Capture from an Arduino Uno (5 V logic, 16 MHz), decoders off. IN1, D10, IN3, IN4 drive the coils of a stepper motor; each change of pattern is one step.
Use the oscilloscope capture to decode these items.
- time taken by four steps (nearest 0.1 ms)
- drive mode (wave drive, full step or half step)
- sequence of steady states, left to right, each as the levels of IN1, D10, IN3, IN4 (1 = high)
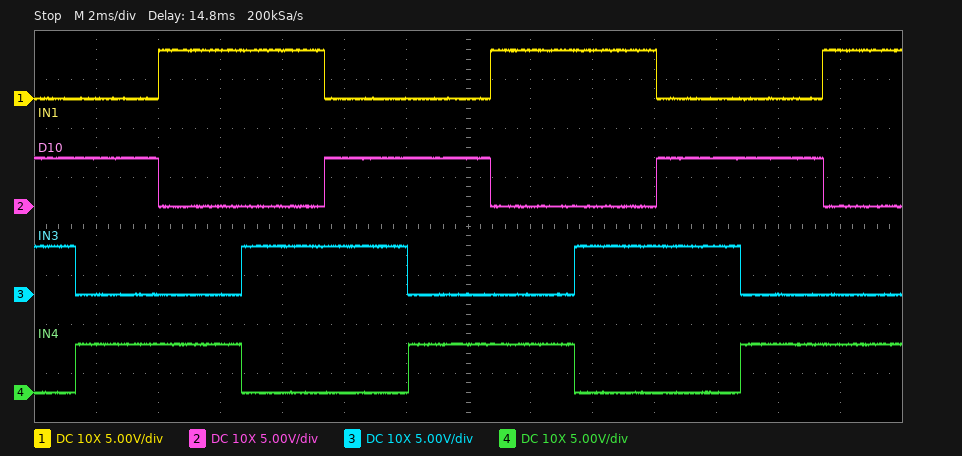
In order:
10.7 ms
full step
0110 0101 1001 1010 0110 0101 1001 1010 0110 0101 1001
